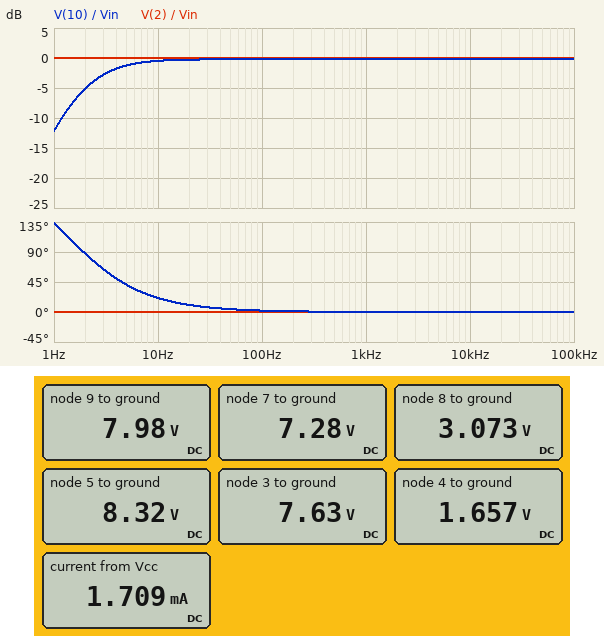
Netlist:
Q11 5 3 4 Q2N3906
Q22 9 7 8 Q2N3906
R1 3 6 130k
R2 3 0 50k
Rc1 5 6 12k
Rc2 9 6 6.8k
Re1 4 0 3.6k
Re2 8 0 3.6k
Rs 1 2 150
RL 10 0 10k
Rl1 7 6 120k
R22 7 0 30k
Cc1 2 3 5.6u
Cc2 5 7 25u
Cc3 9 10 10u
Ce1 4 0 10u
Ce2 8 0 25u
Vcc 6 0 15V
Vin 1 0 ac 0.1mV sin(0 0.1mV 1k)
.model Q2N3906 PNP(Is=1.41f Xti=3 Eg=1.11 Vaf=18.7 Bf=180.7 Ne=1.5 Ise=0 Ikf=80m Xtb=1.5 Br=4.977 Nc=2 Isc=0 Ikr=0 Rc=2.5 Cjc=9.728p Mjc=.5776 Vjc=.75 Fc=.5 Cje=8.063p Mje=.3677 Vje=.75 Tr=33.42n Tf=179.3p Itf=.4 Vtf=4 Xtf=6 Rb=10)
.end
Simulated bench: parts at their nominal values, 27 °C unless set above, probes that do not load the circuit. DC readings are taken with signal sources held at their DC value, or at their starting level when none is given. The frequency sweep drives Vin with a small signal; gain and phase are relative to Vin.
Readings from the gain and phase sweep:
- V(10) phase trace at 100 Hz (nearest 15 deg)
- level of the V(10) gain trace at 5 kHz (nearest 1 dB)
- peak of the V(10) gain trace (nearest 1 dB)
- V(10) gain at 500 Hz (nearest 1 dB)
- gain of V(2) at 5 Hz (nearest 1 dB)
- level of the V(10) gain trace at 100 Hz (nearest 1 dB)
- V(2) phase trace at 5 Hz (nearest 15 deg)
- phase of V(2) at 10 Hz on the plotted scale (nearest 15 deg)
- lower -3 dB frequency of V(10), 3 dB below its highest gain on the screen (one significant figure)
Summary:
0 deg
0 dB
0 dB
0 dB
0 dB
0 dB
0 deg
0 deg
3 Hz
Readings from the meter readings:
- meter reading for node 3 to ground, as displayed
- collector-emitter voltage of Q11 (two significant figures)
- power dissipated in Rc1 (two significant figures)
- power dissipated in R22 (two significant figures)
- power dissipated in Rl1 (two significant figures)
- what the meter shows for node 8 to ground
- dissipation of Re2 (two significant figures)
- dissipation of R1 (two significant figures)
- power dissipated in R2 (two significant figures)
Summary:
7.63 V
6.7 V
3.7 mW
1.8 mW
500 µW
3.073 V
2.6 mW
420 µW
1.2 mW
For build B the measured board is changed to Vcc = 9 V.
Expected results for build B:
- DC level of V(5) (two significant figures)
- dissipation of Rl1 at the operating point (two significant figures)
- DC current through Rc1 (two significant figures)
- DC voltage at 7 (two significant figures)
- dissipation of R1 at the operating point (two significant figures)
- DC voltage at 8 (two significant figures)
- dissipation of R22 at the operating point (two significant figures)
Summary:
5.2 V
190 µW
320 µA
4.3 V
160 µW
1.8 V
610 µW
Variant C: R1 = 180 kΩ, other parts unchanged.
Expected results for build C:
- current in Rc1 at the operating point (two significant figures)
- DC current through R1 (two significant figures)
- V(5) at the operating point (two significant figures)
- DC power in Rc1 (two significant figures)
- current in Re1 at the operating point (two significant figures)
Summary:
590 µA
43 µA
7.9 V
4.2 mW
490 µA
